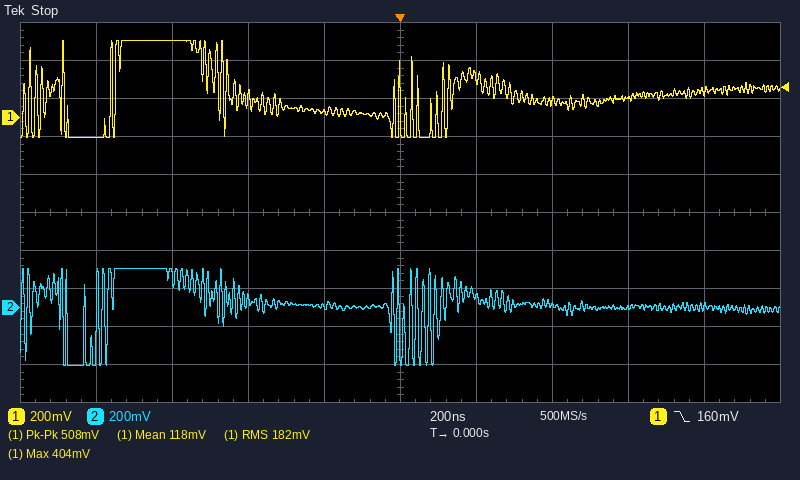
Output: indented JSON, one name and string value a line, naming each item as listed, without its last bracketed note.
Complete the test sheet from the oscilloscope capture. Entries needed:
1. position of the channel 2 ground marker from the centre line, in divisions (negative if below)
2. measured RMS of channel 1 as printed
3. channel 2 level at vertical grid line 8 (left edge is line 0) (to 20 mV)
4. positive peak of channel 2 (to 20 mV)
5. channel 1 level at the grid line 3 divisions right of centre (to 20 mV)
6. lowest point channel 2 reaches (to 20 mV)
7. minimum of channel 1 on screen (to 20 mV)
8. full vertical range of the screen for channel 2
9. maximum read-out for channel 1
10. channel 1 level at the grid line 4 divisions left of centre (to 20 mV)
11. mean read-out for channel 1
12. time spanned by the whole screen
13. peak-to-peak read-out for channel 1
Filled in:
{
  "position of the channel 2 ground marker from the centre line, in divisions": "-2.5 div",
  "measured RMS of channel 1 as printed": "182 mV",
  "channel 2 level at vertical grid line 8 (left edge is line 0)": "0 mV",
  "positive peak of channel 2": "200 mV",
  "channel 1 level at the grid line 3 divisions right of centre": "100 mV",
  "lowest point channel 2 reaches": "-300 mV",
  "minimum of channel 1 on screen": "-100 mV",
  "full vertical range of the screen for channel 2": "2 V",
  "maximum read-out for channel 1": "404 mV",
  "channel 1 level at the grid line 4 divisions left of centre": "-100 mV",
  "mean read-out for channel 1": "118 mV",
  "time spanned by the whole screen": "2 µs",
  "peak-to-peak read-out for channel 1": "508 mV"
}
